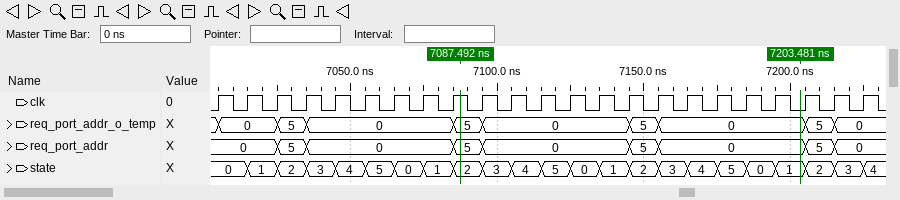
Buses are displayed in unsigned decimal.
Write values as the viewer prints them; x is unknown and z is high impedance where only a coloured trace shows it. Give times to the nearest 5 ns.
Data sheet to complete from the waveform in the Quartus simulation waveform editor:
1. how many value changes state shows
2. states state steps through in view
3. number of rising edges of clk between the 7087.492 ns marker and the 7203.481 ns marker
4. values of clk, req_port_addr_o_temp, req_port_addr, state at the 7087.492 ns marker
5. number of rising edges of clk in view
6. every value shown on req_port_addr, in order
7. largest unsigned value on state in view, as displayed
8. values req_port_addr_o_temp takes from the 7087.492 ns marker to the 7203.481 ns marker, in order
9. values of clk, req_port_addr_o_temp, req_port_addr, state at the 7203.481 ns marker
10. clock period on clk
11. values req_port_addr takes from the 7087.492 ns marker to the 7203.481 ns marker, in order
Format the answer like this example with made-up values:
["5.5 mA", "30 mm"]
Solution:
["22", "0, 1, 2, 3, 4, 5, 0, 1, 2, 3, 4, 5, 0, 1, 2, 3, 4, 5, 0, 1, 2, 3, 4", "11", "clk=1, req_port_addr_o_temp=5, req_port_addr=5, state=2", "23", "0, 5, 0, 5, 0, 5, 0, 5, 0", "5", "5, 0, 5, 0", "clk=0, req_port_addr_o_temp=0, req_port_addr=0, state=1", "10 ns", "5, 0, 5, 0"]
